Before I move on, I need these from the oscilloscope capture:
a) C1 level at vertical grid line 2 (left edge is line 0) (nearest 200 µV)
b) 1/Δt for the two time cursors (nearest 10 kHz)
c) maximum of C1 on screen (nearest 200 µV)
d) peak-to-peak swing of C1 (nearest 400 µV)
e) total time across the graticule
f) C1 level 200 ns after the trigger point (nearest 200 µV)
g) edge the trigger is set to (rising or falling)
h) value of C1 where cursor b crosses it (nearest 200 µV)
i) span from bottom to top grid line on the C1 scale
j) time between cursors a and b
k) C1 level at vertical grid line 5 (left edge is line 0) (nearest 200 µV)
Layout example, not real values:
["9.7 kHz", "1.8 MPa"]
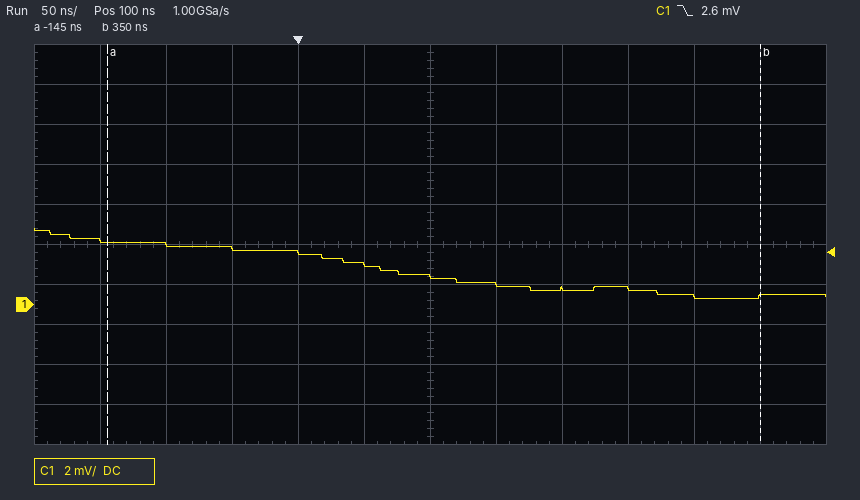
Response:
["3.0 mV", "2.02 MHz", "3.8 mV", "3.6 mV", "600 ns", "800 µV", "falling", "400 µV", "20 mV", "495 ns", "2.0 mV"]
